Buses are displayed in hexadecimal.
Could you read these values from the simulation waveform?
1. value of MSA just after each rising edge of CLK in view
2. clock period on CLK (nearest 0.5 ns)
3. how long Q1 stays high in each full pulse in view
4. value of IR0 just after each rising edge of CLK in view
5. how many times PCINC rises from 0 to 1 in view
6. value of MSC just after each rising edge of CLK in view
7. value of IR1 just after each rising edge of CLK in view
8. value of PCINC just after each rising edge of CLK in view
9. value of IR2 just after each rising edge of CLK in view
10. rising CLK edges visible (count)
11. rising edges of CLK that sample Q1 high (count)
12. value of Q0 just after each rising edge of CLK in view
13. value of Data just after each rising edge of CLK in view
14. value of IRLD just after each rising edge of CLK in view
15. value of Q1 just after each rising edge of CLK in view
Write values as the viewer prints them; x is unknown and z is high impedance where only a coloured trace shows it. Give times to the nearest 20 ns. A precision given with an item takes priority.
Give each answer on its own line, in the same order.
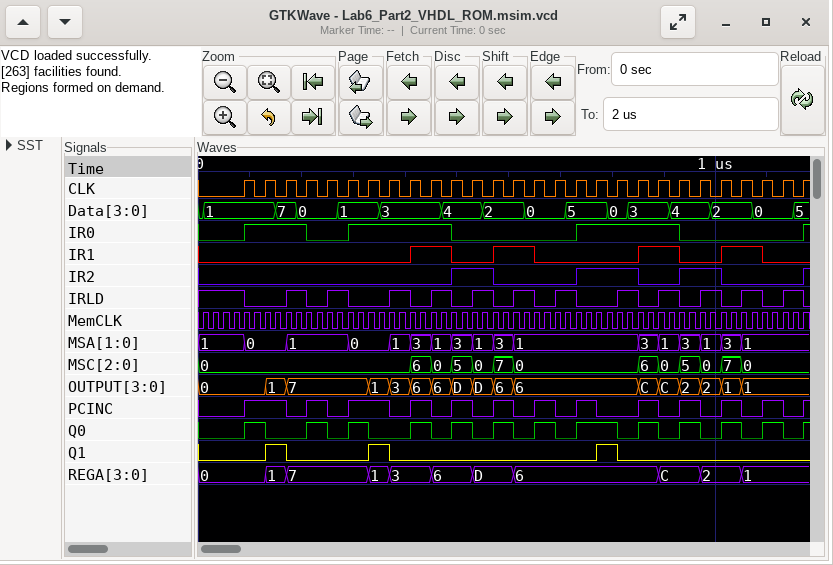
0, 0, 1, 1, 1, 0, 0, 1, 3, 1, 3, 1, 3, 1, 1, 1, 1, 1, 1, 3, 1, 3, 1, 3, 1, 1, 1, 1
40 ns
40 ns, 40 ns, 40 ns
1 1 1 0 0 1 1 1 1 1 0 0 0 0 0 0 1 1 1 1 1 0 0 0 0 0 0 1
13
0, 0, 0, 0, 0, 0, 0, 0, 6, 0, 5, 0, 7, 0, 0, 0, 0, 0, 0, 6, 0, 5, 0, 7, 0, 0, 0, 0
0 0 0 0 0 0 0 0 1 1 0 0 1 1 0 0 0 0 0 1 1 0 0 1 1 0 0 0
1 1 0 1 0 1 1 0 1 0 1 0 1 0 1 0 1 0 0 1 0 1 0 1 0 1 0 1
0 0 0 0 0 0 0 0 0 0 1 1 0 0 0 0 1 1 1 0 0 1 1 0 0 0 0 1
28
3
1 0 0 1 0 1 0 0 1 0 1 0 1 0 1 0 1 1 0 1 0 1 0 1 0 1 0 1
1, 1, 7, 0, 0, 1, 1, 3, 3, 3, 4, 4, 2, 2, 0, 0, 5, 5, 0, 3, 3, 4, 4, 2, 2, 0, 0, 5
0 0 1 0 1 0 0 1 0 1 0 1 0 1 0 1 0 0 1 0 1 0 1 0 1 0 1 0
0 1 0 0 0 0 1 0 0 0 0 0 0 0 0 0 0 1 0 0 0 0 0 0 0 0 0 0
